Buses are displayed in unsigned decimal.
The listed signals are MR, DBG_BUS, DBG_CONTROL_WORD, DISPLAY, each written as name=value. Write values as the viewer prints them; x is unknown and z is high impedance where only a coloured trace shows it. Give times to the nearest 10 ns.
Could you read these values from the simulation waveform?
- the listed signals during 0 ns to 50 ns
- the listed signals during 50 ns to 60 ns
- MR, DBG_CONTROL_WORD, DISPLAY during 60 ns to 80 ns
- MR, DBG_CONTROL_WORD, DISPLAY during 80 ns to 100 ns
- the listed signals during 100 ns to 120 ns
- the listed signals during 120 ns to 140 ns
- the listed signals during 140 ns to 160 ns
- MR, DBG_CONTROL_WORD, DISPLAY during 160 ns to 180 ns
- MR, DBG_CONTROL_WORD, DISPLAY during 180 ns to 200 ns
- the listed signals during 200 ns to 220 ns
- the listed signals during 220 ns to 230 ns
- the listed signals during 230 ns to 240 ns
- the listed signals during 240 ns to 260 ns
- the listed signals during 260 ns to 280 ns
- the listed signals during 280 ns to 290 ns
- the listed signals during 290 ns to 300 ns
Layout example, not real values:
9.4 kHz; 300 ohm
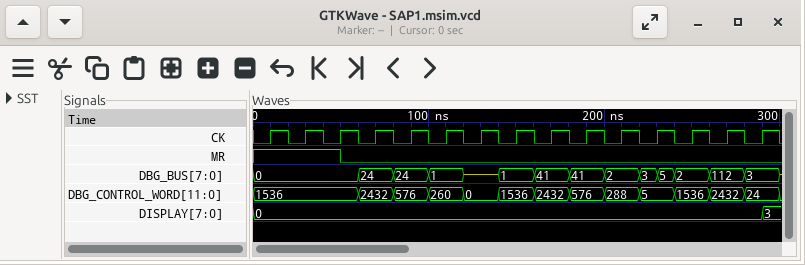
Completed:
MR=1, DBG_BUS=0, DBG_CONTROL_WORD=1536, DISPLAY=0; MR=0, DBG_BUS=0, DBG_CONTROL_WORD=1536, DISPLAY=0; MR=0, DBG_CONTROL_WORD=2432, DISPLAY=0; MR=0, DBG_CONTROL_WORD=576, DISPLAY=0; MR=0, DBG_BUS=1, DBG_CONTROL_WORD=260, DISPLAY=0; MR=0, DBG_BUS=z, DBG_CONTROL_WORD=0, DISPLAY=0; MR=0, DBG_BUS=1, DBG_CONTROL_WORD=1536, DISPLAY=0; MR=0, DBG_CONTROL_WORD=2432, DISPLAY=0; MR=0, DBG_CONTROL_WORD=576, DISPLAY=0; MR=0, DBG_BUS=2, DBG_CONTROL_WORD=288, DISPLAY=0; MR=0, DBG_BUS=3, DBG_CONTROL_WORD=5, DISPLAY=0; MR=0, DBG_BUS=5, DBG_CONTROL_WORD=5, DISPLAY=0; MR=0, DBG_BUS=2, DBG_CONTROL_WORD=1536, DISPLAY=0; MR=0, DBG_BUS=112, DBG_CONTROL_WORD=2432, DISPLAY=0; MR=0, DBG_BUS=3, DBG_CONTROL_WORD=24, DISPLAY=0; MR=0, DBG_BUS=3, DBG_CONTROL_WORD=24, DISPLAY=3
